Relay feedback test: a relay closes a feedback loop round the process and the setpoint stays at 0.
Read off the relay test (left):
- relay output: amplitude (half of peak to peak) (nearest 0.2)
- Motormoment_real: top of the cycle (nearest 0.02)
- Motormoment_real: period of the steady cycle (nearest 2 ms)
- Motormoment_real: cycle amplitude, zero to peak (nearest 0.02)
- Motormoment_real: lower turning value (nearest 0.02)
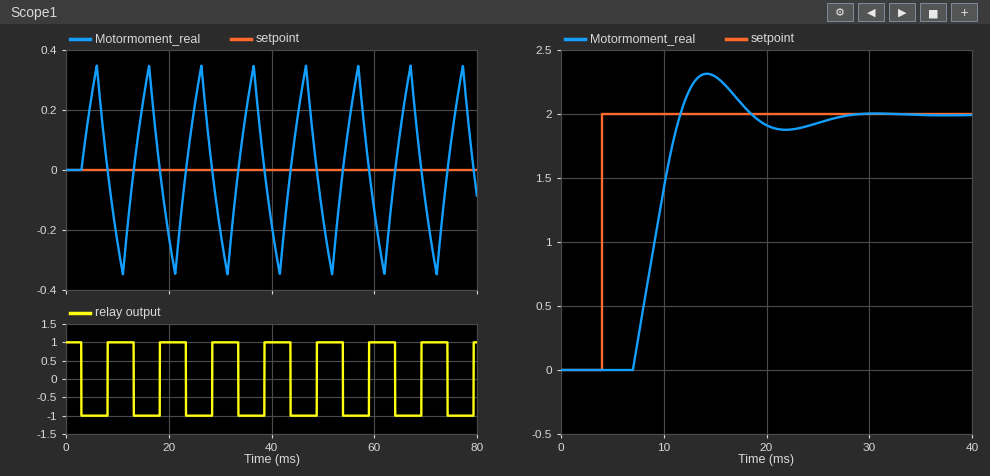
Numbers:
1.0
0.34
10 ms
0.34
-0.34
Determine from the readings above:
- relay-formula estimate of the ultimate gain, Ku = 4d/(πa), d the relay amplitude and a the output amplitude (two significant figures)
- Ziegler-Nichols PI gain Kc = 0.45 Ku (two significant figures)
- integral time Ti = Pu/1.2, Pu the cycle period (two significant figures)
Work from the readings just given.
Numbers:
3.7
1.7
8.3 ms
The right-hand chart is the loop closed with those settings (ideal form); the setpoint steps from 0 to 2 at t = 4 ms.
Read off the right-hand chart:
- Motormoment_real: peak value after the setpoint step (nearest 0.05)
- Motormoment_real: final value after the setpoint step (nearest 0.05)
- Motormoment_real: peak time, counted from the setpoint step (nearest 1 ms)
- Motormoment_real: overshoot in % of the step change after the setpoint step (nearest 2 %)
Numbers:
2.30
2.00
10 ms
16 %
